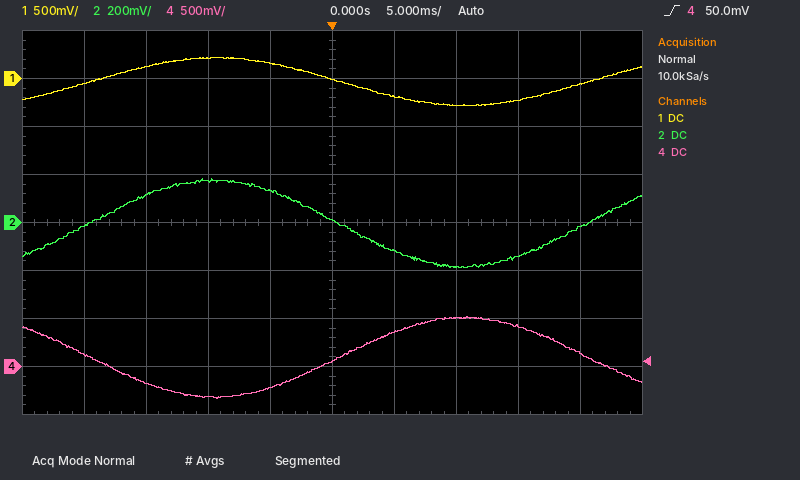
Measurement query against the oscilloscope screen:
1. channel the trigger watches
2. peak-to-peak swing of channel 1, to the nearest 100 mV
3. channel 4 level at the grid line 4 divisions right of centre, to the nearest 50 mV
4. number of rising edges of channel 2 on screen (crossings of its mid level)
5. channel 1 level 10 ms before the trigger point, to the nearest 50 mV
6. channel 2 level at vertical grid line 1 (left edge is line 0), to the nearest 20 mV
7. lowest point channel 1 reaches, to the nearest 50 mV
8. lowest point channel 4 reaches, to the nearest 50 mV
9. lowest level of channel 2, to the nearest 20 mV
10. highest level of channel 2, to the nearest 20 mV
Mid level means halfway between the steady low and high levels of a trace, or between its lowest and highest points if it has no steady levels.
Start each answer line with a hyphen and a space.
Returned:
- channel 4
- 500 mV
- 150 mV
- 2
- 200 mV
- -20 mV
- -300 mV
- -350 mV
- -180 mV
- 180 mV
